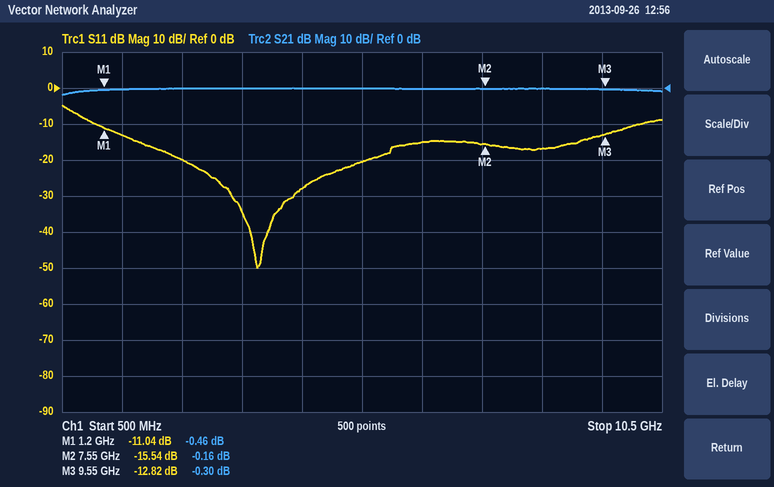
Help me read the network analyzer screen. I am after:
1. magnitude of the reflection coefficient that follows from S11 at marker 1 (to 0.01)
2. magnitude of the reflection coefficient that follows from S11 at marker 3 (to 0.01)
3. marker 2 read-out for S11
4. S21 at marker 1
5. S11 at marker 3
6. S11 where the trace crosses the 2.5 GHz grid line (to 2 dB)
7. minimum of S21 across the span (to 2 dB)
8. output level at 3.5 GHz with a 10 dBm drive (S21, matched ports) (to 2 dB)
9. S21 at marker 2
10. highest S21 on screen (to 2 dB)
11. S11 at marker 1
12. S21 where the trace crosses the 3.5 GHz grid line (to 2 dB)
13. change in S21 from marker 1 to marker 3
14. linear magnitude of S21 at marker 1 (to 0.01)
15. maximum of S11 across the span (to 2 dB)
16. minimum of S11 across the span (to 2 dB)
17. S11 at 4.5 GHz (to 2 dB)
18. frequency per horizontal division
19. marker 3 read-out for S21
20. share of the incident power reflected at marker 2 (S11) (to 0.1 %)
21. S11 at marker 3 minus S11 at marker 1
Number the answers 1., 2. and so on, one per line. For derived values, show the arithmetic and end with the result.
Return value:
1. 10^(-11.04/20) ≈ 0.28
2. 10^(-12.82/20) ≈ 0.23
3. -15.54 dB
4. -0.46 dB
5. -12.82 dB
6. -20 dB
7. -2 dB
8. 10 dBm + (0 dB) = 10 dBm
9. -0.16 dB
10. 0 dB
11. -11.04 dB
12. 0 dB
13. -0.3 − (-0.46) = 0.16 dB
14. 10^(-0.46/20) ≈ 0.95
15. -4 dB
16. -50 dB
17. -28 dB
18. 1 GHz
19. -0.30 dB
20. 10^(-15.54/10) ≈ 2.8 %
21. -12.82 − (-11.04) = -1.78 dB
